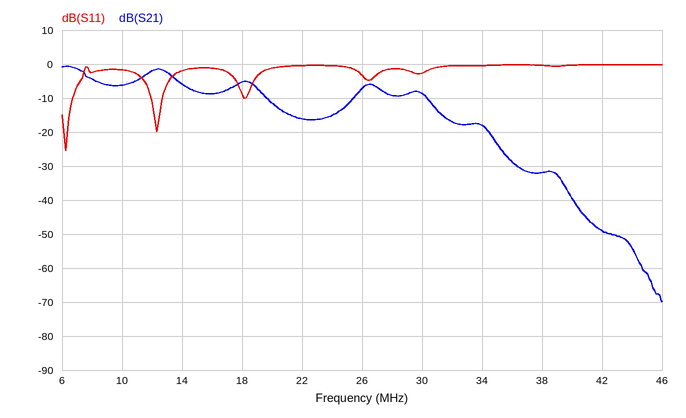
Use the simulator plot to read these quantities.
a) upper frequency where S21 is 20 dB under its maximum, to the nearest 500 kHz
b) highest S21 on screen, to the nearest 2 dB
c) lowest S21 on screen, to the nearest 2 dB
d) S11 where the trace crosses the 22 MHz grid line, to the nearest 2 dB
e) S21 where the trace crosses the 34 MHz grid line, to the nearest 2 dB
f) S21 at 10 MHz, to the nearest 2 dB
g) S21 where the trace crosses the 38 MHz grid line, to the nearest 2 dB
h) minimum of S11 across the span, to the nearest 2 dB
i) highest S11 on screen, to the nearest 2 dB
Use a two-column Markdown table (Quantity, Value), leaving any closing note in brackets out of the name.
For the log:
| Quantity | Value |
|---|---|
| upper frequency where S21 is 20 dB under its maximum, to the nearest 500 kHz | 34.5 MHz |
| highest S21 on screen, to the nearest 2 dB | 0 dB |
| lowest S21 on screen, to the nearest 2 dB | -70 dB |
| S11 where the trace crosses the 22 MHz grid line, to the nearest 2 dB | 0 dB |
| S21 where the trace crosses the 34 MHz grid line, to the nearest 2 dB | -18 dB |
| S21 at 10 MHz, to the nearest 2 dB | -6 dB |
| S21 where the trace crosses the 38 MHz grid line, to the nearest 2 dB | -32 dB |
| minimum of S11 across the span, to the nearest 2 dB | -26 dB |
| highest S11 on screen, to the nearest 2 dB | 0 dB |
